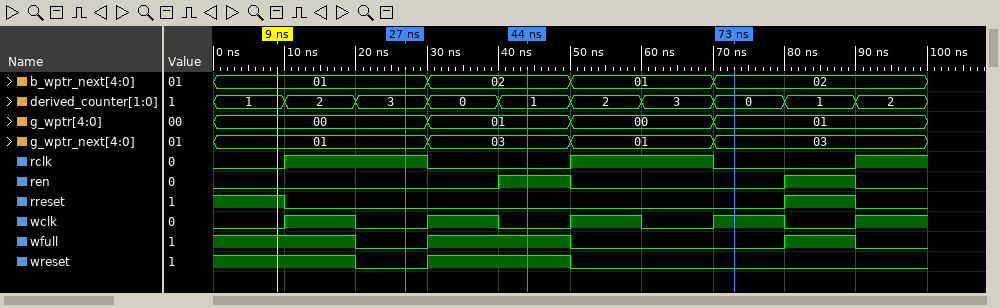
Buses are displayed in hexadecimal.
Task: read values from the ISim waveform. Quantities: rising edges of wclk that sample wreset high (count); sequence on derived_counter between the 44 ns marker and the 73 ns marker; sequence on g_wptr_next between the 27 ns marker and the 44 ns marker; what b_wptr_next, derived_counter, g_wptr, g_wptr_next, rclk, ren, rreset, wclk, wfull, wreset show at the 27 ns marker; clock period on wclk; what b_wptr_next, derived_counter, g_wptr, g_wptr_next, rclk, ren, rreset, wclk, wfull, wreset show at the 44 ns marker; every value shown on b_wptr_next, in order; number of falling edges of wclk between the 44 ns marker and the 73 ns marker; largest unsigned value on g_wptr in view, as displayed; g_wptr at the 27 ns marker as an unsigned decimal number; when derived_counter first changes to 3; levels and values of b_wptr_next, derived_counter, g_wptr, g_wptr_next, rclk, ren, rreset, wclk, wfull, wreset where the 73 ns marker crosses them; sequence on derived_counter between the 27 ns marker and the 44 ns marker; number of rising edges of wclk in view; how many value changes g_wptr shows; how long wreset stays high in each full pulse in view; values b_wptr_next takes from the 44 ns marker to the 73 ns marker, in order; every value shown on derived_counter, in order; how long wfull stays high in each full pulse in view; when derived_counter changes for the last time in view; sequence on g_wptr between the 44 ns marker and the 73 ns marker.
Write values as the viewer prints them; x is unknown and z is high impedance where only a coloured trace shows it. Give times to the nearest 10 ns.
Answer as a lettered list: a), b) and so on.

a) 2
b) 1, 2, 3, 0
c) 01, 03
d) b_wptr_next=01, derived_counter=3, g_wptr=00, g_wptr_next=01, rclk=1, ren=0, rreset=0, wclk=0, wfull=0, wreset=0
e) 20 ns
f) b_wptr_next=02, derived_counter=1, g_wptr=01, g_wptr_next=03, rclk=0, ren=1, rreset=0, wclk=0, wfull=1, wreset=1
g) 01, 02, 01, 02
h) 1
i) 01
j) 0
k) 20 ns
l) b_wptr_next=02, derived_counter=0, g_wptr=01, g_wptr_next=03, rclk=0, ren=0, rreset=0, wclk=1, wfull=0, wreset=0
m) 3, 0, 1
n) 5
o) 3
p) 20 ns
q) 02, 01, 02
r) 1, 2, 3, 0, 1, 2, 3, 0, 1, 2
s) 20 ns, 10 ns
t) 90 ns
u) 01, 00, 01
